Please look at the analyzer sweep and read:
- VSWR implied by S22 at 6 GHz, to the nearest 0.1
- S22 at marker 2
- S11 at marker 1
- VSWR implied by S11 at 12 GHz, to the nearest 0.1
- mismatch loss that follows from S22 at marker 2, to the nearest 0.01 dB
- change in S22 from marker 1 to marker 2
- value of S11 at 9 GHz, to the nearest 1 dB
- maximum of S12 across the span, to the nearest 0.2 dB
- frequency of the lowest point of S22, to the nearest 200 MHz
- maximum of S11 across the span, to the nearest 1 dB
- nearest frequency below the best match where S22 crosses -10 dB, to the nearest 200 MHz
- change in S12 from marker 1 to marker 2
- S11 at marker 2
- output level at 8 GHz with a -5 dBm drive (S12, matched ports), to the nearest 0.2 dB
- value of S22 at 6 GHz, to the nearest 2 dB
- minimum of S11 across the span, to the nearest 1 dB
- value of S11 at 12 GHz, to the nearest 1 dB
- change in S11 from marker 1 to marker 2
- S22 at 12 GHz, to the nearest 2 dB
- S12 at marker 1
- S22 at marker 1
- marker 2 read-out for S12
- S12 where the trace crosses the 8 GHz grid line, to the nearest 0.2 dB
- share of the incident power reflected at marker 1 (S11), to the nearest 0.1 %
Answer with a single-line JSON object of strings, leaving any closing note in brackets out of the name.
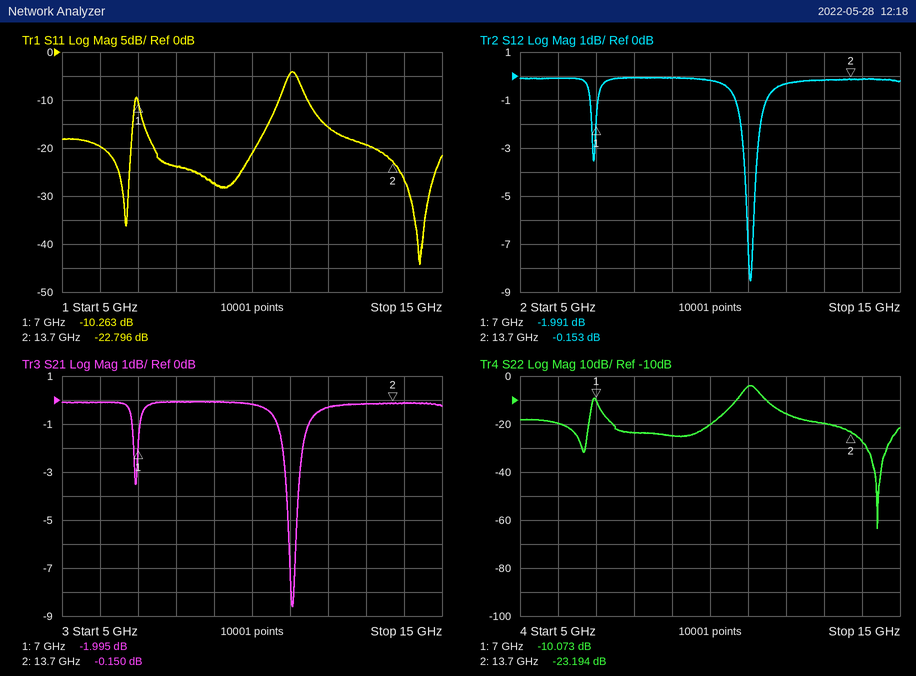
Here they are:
{"VSWR implied by S22 at 6 GHz, to the nearest 0.1": "1.2", "S22 at marker 2": "-23.194 dB", "S11 at marker 1": "-10.263 dB", "VSWR implied by S11 at 12 GHz, to the nearest 0.1": "1.4", "mismatch loss that follows from S22 at marker 2, to the nearest 0.01 dB": "0.02 dB", "change in S22 from marker 1 to marker 2": "-13.121 dB", "value of S11 at 9 GHz, to the nearest 1 dB": "-27 dB", "maximum of S12 across the span, to the nearest 0.2 dB": "0.0 dB", "frequency of the lowest point of S22, to the nearest 200 MHz": "14.4 GHz", "maximum of S11 across the span, to the nearest 1 dB": "-4 dB", "nearest frequency below the best match where S22 crosses -10 dB, to the nearest 200 MHz": "11.4 GHz", "change in S12 from marker 1 to marker 2": "1.838 dB", "S11 at marker 2": "-22.796 dB", "output level at 8 GHz with a -5 dBm drive (S12, matched ports), to the nearest 0.2 dB": "-5.0 dBm", "value of S22 at 6 GHz, to the nearest 2 dB": "-20 dB", "minimum of S11 across the span, to the nearest 1 dB": "-44 dB", "value of S11 at 12 GHz, to the nearest 1 dB": "-16 dB", "change in S11 from marker 1 to marker 2": "-12.533 dB", "S22 at 12 GHz, to the nearest 2 dB": "-16 dB", "S12 at marker 1": "-1.991 dB", "S22 at marker 1": "-10.073 dB", "marker 2 read-out for S12": "-0.153 dB", "S12 where the trace crosses the 8 GHz grid line, to the nearest 0.2 dB": "0.0 dB", "share of the incident power reflected at marker 1 (S11), to the nearest 0.1 %": "9.4 %"}
